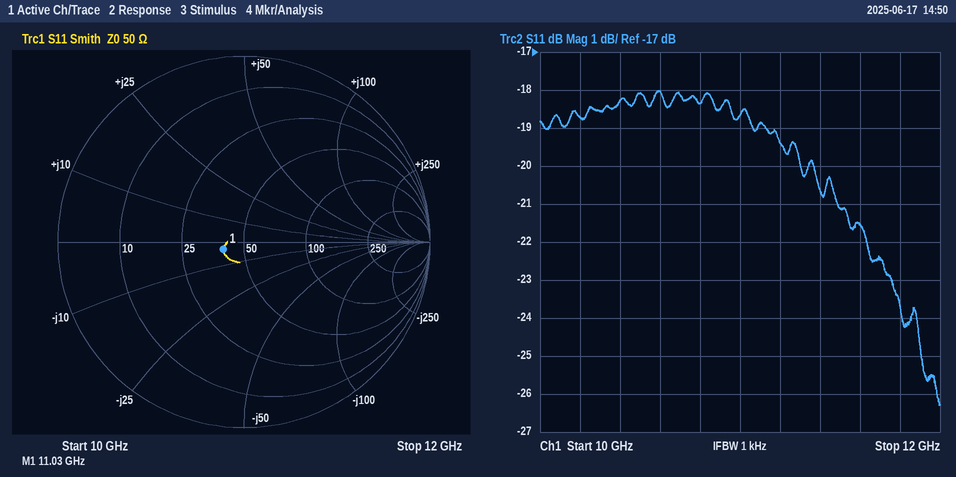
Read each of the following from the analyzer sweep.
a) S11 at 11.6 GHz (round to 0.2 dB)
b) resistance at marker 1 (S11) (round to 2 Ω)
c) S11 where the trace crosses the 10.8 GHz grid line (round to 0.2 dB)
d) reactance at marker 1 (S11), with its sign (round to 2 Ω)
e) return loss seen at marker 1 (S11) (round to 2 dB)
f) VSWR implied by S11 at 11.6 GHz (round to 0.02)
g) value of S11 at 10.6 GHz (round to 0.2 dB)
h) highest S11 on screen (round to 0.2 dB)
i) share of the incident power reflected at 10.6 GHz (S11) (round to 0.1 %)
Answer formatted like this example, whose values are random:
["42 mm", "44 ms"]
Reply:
["-21.6 dB", "40 Ω", "-18.4 dB", "-4 Ω", "18 dB", "1.18", "-18.0 dB", "-18.0 dB", "1.6 %"]
